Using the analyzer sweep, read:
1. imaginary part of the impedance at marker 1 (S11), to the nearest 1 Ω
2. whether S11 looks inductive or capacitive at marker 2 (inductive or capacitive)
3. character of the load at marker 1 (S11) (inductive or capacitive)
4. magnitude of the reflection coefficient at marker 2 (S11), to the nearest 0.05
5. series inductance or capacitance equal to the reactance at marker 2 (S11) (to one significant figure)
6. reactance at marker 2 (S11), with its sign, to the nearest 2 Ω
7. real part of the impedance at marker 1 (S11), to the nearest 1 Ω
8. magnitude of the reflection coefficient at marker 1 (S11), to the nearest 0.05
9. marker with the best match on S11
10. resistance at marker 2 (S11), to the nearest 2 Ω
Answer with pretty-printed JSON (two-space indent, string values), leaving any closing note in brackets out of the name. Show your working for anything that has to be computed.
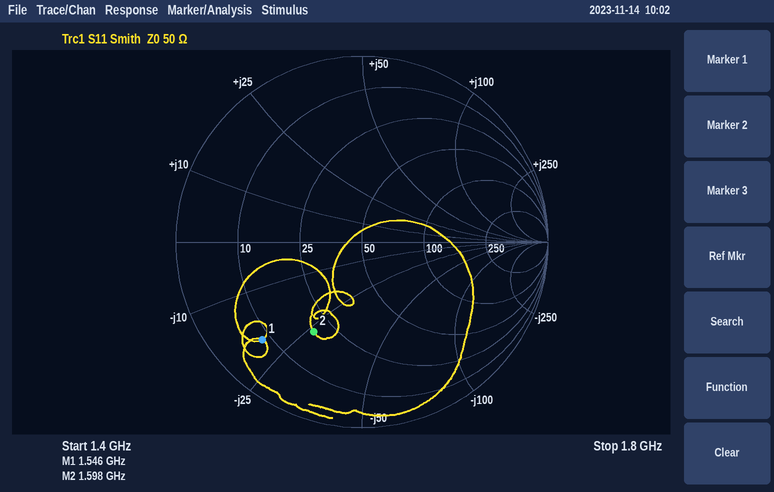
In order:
{
  "imaginary part of the impedance at marker 1 (S11), to the nearest 1 Ω": "-20 Ω",
  "whether S11 looks inductive or capacitive at marker 2": "capacitive",
  "character of the load at marker 1 (S11)": "capacitive",
  "magnitude of the reflection coefficient at marker 2 (S11), to the nearest 0.05": "0.55",
  "series inductance or capacitance equal to the reactance at marker 2 (S11)": "C = 1/(2π × 1.598 GHz × 26 Ω) ≈ 4 pF",
  "reactance at marker 2 (S11), with its sign, to the nearest 2 Ω": "-26 Ω",
  "real part of the impedance at marker 1 (S11), to the nearest 1 Ω": "8 Ω",
  "magnitude of the reflection coefficient at marker 1 (S11), to the nearest 0.05": "0.75",
  "marker with the best match on S11": "marker 2",
  "resistance at marker 2 (S11), to the nearest 2 Ω": "20 Ω"
}
